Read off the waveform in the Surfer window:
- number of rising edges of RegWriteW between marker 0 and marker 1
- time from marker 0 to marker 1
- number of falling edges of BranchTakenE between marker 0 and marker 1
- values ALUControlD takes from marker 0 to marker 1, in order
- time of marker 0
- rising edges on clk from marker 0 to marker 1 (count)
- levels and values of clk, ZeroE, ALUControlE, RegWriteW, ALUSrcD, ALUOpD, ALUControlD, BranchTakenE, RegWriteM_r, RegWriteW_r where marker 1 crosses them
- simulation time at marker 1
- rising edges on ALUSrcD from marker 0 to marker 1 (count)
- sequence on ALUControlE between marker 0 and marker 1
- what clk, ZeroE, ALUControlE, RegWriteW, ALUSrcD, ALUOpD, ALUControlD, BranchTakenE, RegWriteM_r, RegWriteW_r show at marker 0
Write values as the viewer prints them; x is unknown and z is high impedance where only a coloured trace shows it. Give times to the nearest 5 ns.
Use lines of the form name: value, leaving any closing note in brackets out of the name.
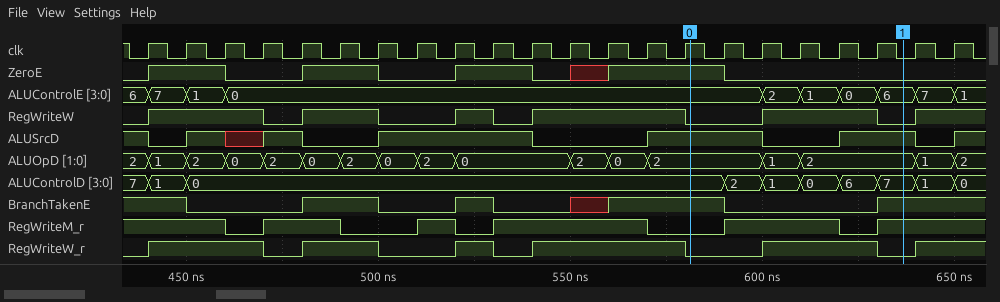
number of rising edges of RegWriteW between marker 0 and marker 1: 1
time from marker 0 to marker 1: 55 ns
number of falling edges of BranchTakenE between marker 0 and marker 1: 1
values ALUControlD takes from marker 0 to marker 1, in order: 0, 2, 1, 0, 6, 7
time of marker 0: 580 ns
rising edges on clk from marker 0 to marker 1: 5
levels and values of clk, ZeroE, ALUControlE, RegWriteW, ALUSrcD, ALUOpD, ALUControlD, BranchTakenE, RegWriteM_r, RegWriteW_r where marker 1 crosses them: clk=0, ZeroE=0, ALUControlE=6, RegWriteW=0, ALUSrcD=1, ALUOpD=2, ALUControlD=7, BranchTakenE=1, RegWriteM_r=1, RegWriteW_r=0
simulation time at marker 1: 635 ns
rising edges on ALUSrcD from marker 0 to marker 1: 1
sequence on ALUControlE between marker 0 and marker 1: 0, 2, 1, 0, 6
what clk, ZeroE, ALUControlE, RegWriteW, ALUSrcD, ALUOpD, ALUControlD, BranchTakenE, RegWriteM_r, RegWriteW_r show at marker 0: clk=1, ZeroE=1, ALUControlE=0, RegWriteW=0, ALUSrcD=1, ALUOpD=2, ALUControlD=0, BranchTakenE=1, RegWriteM_r=0, RegWriteW_r=0
